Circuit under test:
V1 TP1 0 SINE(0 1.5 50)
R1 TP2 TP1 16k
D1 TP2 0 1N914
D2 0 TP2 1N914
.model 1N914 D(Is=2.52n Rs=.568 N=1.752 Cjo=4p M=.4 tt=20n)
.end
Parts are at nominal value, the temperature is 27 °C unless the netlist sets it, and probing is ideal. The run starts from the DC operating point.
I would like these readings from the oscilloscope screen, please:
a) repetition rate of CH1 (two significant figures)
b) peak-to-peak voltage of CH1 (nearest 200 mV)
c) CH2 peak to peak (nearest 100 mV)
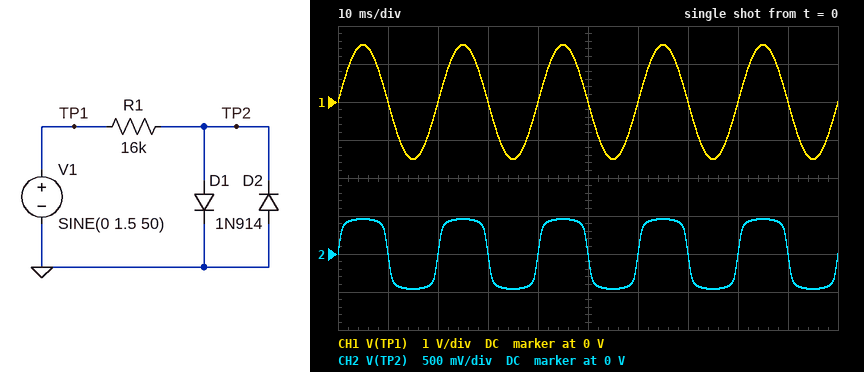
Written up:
50 Hz
3.0 V
900 mV
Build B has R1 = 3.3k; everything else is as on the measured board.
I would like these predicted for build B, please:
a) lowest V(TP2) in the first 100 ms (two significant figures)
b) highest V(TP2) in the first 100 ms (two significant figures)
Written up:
-530 mV
530 mV
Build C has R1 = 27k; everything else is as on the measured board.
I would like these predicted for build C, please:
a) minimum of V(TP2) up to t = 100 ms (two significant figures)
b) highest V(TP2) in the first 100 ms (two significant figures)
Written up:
-440 mV
440 mV
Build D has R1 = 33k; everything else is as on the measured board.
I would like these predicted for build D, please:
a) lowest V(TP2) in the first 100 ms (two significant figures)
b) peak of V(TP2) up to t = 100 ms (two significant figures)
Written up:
-430 mV
430 mV
